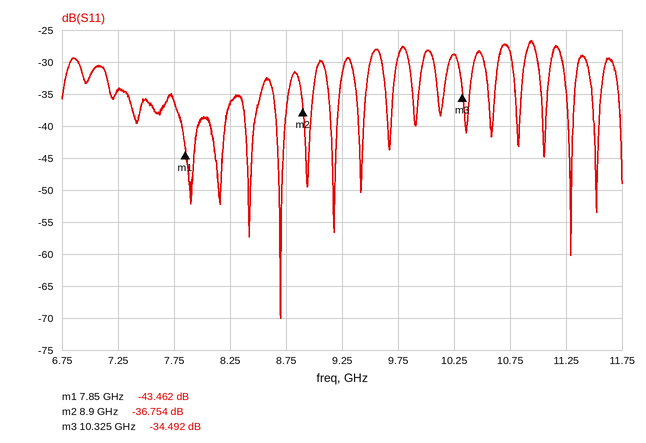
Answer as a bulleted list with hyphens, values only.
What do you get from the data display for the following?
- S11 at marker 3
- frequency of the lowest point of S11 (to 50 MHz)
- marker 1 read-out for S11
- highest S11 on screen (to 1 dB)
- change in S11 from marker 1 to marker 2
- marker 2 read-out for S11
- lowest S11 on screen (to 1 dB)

- -34.492 dB
- 8.70 GHz
- -43.462 dB
- -27 dB
- 6.708 dB
- -36.754 dB
- -70 dB
